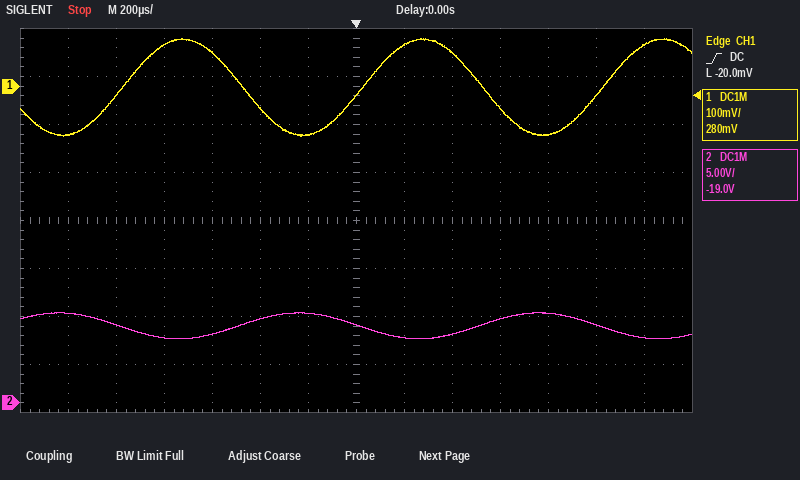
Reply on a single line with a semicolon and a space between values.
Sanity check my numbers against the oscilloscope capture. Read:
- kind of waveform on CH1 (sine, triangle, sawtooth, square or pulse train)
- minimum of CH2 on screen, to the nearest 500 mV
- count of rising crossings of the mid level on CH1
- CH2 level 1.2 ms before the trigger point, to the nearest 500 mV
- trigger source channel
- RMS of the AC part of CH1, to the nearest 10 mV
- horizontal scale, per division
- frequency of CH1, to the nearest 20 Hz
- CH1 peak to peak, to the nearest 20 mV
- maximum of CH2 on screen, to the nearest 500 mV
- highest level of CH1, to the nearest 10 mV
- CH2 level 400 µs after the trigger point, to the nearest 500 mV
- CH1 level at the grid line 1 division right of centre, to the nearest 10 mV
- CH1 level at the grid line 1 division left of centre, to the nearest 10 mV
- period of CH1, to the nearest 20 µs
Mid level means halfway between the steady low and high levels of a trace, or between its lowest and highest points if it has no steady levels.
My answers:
sine; 6.5 V; 3; 9.5 V; CH1; 70 mV; 200 µs; 1.00 kHz; 200 mV; 9.5 V; 100 mV; 7.0 V; 90 mV; -100 mV; 1.00 ms
